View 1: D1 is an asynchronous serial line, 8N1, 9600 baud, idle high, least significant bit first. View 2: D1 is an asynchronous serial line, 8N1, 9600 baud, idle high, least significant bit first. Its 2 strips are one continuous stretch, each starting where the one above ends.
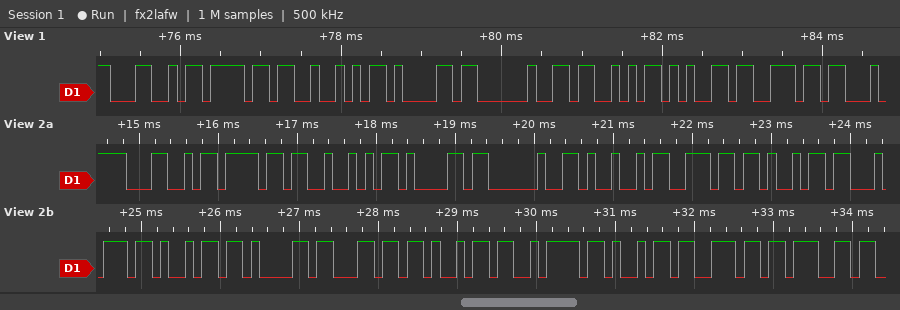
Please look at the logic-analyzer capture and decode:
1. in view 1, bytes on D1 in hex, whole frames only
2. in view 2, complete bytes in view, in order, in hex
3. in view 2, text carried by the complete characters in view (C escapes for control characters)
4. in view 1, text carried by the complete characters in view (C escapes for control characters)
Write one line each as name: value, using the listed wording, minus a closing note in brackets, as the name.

in view 1, bytes on D1 in hex, whole frames only: 4C 6F 52 61 20 53 65 6E
in view 2, complete bytes in view, in order, in hex: 4C 6F 52 61 20 49 6E 69 74 69 61 6C 69 7A 69 6E 67
in view 2, text carried by the complete characters in view: "LoRa Initializing"
in view 1, text carried by the complete characters in view: "LoRa Sen"
